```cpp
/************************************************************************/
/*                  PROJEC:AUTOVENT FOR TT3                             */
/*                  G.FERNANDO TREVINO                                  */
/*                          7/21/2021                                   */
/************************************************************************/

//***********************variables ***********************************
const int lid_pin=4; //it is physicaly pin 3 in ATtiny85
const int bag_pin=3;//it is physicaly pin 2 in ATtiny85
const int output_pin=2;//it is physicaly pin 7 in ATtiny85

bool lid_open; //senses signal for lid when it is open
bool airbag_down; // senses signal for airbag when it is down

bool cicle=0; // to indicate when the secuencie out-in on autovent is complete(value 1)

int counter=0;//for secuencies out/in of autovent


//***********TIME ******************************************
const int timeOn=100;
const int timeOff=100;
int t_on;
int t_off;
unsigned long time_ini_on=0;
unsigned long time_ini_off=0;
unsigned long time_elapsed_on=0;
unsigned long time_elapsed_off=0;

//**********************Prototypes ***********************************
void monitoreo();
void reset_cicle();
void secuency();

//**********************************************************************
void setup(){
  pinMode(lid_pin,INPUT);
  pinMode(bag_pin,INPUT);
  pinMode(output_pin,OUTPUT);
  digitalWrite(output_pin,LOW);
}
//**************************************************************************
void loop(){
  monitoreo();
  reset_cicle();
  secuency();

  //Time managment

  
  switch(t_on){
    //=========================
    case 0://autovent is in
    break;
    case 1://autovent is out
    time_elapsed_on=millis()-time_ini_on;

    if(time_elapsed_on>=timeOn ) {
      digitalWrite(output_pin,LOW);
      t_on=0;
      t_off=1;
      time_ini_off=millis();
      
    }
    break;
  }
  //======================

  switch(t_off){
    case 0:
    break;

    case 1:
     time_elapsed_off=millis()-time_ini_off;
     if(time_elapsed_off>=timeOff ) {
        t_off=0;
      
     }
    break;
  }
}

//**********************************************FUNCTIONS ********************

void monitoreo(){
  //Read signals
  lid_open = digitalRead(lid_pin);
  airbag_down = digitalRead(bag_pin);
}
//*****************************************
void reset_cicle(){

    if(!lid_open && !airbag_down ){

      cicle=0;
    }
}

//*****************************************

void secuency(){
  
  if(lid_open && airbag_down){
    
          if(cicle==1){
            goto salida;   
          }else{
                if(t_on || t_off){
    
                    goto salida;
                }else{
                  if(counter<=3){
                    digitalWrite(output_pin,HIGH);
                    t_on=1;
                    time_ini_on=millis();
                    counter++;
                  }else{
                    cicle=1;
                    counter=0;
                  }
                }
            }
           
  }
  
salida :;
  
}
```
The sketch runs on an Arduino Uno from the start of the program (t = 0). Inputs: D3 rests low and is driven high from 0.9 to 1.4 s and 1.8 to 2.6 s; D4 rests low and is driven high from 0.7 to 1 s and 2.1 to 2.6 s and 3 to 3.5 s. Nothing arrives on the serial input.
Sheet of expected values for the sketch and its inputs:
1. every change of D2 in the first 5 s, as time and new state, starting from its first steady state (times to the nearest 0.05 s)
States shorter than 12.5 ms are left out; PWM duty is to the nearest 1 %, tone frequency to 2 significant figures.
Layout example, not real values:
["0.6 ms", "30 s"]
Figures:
["0 s low; 0.9 s high; 1 s low; 2.1 s high; 2.2 s low; 2.3 s high; 2.4 s low; 2.5 s high; 2.6 s low"]
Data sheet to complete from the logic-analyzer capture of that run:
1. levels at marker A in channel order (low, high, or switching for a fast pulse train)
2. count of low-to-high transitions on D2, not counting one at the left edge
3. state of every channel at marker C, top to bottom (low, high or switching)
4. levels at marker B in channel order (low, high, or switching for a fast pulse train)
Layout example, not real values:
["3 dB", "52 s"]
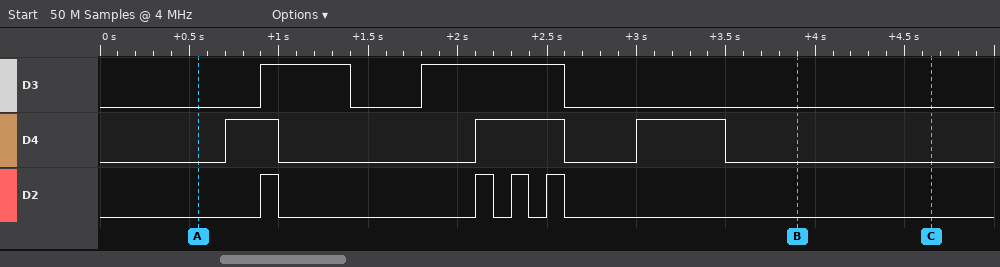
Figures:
["D3 low, D4 low, D2 low", "4", "D3 low, D4 low, D2 low", "D3 low, D4 low, D2 low"]
